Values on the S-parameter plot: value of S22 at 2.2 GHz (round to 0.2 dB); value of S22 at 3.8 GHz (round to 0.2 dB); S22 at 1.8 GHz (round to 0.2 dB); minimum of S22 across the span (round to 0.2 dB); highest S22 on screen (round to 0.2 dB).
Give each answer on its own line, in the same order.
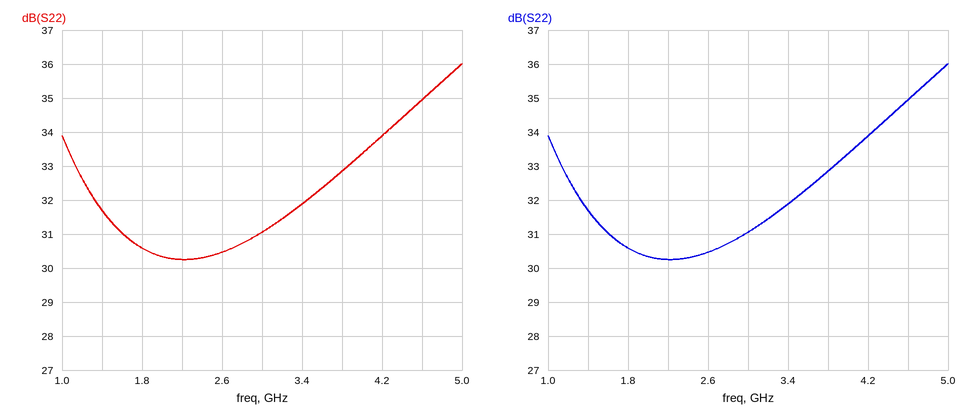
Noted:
30.2 dB
32.8 dB
30.6 dB
30.2 dB
36.0 dB
